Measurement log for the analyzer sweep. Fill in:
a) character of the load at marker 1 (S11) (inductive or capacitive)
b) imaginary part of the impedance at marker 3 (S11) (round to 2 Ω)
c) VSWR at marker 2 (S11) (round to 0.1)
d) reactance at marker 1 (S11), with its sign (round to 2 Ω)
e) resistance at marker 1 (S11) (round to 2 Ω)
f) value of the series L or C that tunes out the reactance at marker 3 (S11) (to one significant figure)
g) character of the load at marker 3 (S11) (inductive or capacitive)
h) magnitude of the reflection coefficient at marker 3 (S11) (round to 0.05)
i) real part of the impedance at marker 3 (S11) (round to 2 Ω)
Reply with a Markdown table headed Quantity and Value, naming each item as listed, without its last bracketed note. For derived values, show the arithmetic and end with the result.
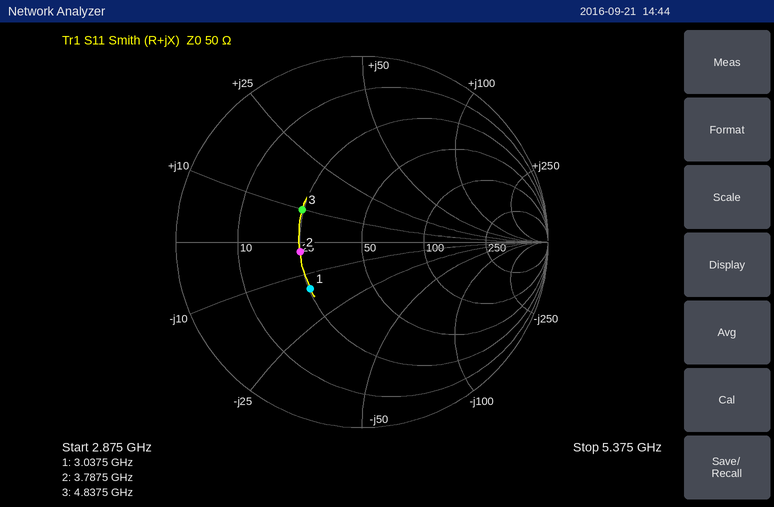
| Quantity | Value |
|---|---|
| character of the load at marker 1 (S11) | capacitive |
| imaginary part of the impedance at marker 3 (S11) | +10 Ω |
| VSWR at marker 2 (S11) | 2.0 |
| reactance at marker 1 (S11), with its sign | -14 Ω |
| resistance at marker 1 (S11) | 26 Ω |
| value of the series L or C that tunes out the reactance at marker 3 (S11) | C = 1/(2π × 4.8375 GHz × 10 Ω) ≈ 3 pF |
| character of the load at marker 3 (S11) | inductive |
| magnitude of the reflection coefficient at marker 3 (S11) | 0.35 |
| real part of the impedance at marker 3 (S11) | 24 Ω |
